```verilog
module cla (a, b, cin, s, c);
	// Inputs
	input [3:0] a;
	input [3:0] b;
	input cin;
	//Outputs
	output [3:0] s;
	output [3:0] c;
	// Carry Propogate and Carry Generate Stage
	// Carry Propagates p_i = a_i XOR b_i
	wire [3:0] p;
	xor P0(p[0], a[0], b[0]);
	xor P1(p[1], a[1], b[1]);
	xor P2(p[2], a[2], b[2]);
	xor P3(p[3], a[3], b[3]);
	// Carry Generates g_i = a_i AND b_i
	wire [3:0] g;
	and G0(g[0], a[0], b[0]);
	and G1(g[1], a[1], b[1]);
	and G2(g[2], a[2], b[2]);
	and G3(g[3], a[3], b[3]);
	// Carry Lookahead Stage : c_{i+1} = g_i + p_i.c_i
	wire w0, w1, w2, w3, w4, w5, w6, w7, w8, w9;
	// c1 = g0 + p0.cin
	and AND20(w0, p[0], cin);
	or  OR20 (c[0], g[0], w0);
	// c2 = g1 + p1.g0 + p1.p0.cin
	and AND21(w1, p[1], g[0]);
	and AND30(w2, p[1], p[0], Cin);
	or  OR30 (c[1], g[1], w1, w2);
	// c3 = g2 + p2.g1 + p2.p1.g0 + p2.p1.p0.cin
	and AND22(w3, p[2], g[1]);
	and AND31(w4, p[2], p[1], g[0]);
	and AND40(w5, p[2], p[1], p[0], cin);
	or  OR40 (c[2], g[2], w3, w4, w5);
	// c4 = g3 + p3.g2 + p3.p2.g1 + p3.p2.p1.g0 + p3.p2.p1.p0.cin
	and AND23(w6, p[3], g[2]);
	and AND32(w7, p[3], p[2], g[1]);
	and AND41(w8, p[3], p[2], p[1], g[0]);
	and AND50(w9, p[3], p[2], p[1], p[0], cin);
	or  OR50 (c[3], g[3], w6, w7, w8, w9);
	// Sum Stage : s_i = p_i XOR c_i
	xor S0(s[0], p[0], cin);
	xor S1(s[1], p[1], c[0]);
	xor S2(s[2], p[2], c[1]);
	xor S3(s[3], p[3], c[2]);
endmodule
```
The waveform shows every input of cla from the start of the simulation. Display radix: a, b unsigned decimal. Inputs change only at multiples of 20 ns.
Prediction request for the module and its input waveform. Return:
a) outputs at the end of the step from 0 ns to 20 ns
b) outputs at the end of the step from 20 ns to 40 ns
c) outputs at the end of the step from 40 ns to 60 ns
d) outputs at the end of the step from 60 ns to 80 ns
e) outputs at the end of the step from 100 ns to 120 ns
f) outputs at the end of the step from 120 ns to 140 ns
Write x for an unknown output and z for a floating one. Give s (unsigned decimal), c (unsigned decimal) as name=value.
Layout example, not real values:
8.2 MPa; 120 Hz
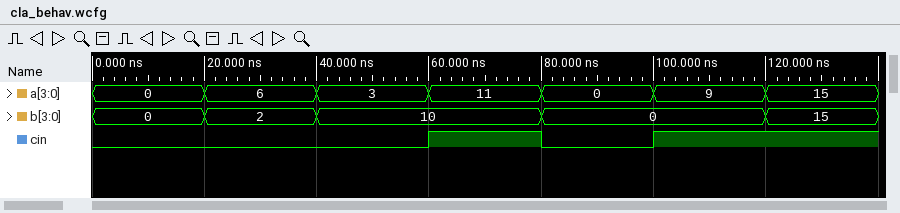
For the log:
s=0, c=0; s=8, c=6; s=13, c=2; s=6, c=11; s=10, c=1; s=15, c=15
